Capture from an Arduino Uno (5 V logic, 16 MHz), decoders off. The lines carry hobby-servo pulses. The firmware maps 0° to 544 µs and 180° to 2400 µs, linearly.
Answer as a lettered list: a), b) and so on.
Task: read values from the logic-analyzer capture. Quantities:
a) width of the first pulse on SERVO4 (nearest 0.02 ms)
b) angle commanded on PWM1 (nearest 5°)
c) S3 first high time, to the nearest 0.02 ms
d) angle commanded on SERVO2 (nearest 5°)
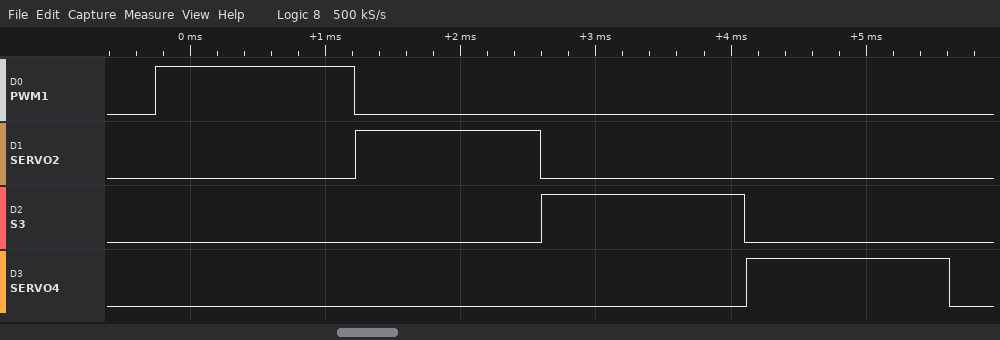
a) 1.50 ms
b) 90°
c) 1.50 ms
d) 80°
